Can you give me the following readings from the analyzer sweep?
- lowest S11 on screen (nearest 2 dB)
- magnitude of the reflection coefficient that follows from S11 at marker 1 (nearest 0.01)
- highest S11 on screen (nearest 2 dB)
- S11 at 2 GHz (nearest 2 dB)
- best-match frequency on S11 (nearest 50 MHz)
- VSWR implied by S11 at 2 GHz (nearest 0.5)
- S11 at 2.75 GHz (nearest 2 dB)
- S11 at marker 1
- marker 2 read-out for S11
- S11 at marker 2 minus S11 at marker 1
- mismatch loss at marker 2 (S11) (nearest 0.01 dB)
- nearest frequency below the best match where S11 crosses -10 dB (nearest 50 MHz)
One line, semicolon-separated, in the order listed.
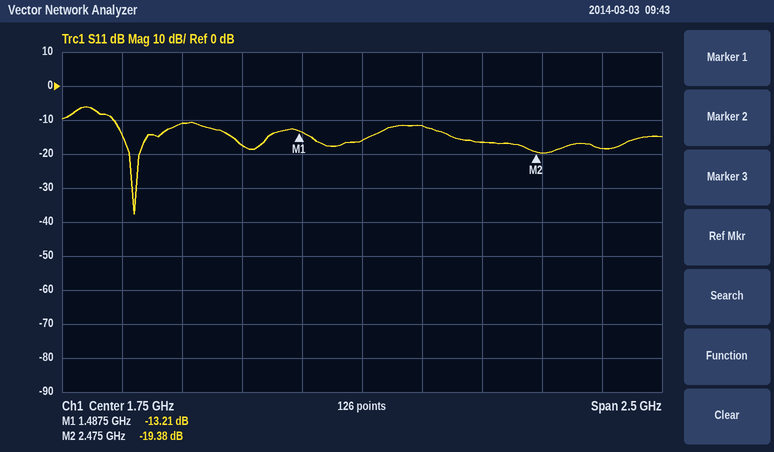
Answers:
-38 dB; 0.22; -6 dB; -12 dB; 800 MHz; 1.5; -18 dB; -13.21 dB; -19.38 dB; -6.17 dB; 0.05 dB; 700 MHz
